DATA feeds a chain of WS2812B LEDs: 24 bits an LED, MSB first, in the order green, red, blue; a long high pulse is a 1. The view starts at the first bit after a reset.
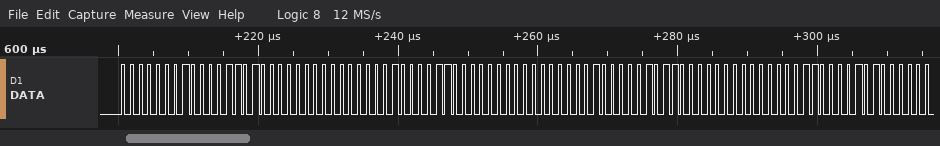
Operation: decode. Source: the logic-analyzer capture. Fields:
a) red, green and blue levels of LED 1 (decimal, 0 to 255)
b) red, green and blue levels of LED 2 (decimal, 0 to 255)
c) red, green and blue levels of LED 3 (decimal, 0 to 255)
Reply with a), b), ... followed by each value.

a) 13, 1, 0
b) 12, 1, 0
c) 11, 2, 0
